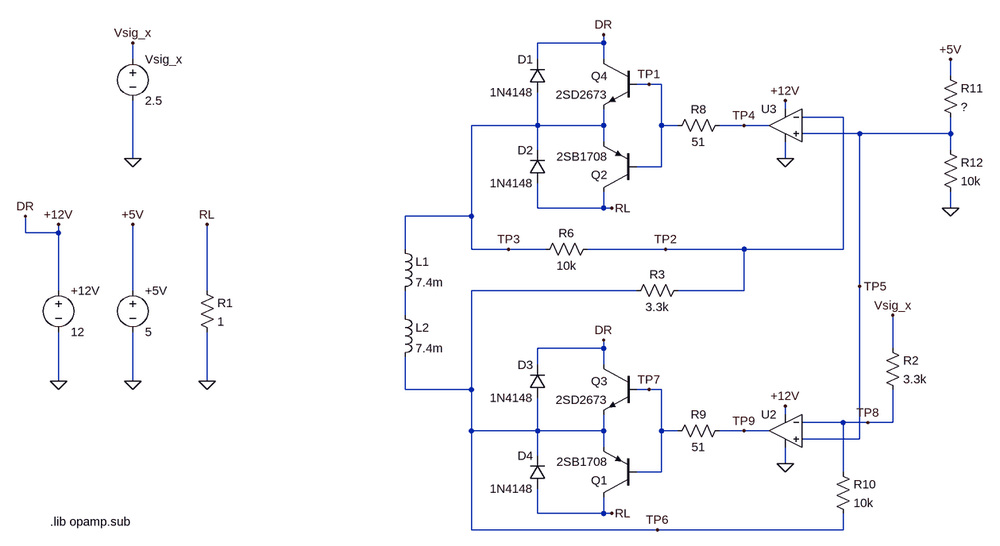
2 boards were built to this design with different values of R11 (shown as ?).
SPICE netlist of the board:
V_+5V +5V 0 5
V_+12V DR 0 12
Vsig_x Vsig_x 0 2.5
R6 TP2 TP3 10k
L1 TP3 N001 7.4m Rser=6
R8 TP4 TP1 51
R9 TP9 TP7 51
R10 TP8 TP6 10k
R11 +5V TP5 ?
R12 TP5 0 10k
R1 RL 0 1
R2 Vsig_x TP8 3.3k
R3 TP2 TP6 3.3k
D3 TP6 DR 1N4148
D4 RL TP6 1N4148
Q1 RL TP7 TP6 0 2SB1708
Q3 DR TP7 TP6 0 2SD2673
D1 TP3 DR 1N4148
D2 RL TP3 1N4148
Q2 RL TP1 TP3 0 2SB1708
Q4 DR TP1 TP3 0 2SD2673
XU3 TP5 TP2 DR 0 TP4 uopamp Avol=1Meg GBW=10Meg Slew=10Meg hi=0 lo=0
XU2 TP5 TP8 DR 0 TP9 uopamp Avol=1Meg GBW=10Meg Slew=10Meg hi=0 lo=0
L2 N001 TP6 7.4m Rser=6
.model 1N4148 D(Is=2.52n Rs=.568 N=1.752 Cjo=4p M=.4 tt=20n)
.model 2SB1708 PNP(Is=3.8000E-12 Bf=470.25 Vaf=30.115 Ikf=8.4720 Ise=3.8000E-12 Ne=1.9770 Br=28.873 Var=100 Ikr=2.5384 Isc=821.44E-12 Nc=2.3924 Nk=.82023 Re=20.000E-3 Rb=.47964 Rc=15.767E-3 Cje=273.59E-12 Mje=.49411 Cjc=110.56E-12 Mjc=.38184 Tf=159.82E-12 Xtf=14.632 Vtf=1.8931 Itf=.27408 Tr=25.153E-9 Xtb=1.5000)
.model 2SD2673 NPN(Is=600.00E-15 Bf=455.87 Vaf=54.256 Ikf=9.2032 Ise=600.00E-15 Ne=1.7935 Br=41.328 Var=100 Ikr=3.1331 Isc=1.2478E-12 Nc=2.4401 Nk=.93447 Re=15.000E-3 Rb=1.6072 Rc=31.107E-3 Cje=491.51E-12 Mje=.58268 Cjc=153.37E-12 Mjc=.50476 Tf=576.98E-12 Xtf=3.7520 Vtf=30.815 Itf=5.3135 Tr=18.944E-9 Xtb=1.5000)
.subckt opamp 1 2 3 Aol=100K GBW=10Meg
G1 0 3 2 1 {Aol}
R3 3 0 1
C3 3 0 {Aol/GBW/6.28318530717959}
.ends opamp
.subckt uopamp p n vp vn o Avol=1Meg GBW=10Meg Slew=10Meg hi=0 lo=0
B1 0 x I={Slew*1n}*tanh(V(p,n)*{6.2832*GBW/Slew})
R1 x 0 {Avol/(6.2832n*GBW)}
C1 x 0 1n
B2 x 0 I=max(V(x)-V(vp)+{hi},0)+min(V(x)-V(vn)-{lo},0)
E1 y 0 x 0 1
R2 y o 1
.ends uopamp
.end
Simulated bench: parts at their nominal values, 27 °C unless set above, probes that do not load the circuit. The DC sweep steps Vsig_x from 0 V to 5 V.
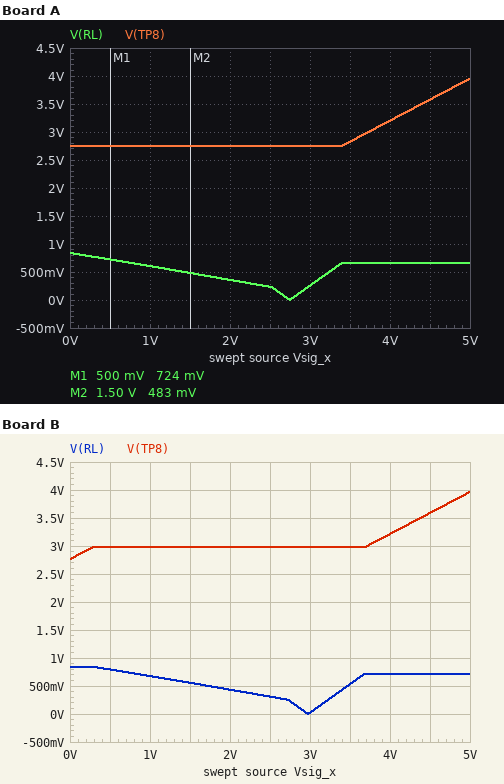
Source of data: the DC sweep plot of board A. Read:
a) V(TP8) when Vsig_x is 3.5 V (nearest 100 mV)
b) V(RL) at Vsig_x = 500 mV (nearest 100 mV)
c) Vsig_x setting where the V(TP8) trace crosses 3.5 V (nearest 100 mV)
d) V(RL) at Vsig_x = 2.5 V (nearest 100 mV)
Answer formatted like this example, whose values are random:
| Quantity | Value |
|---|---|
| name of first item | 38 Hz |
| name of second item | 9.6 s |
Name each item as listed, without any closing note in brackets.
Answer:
| Quantity | Value |
|---|---|
| V(TP8) when Vsig_x is 3.5 V | 2.8 V |
| V(RL) at Vsig_x = 500 mV | 700 mV |
| Vsig_x setting where the V(TP8) trace crosses 3.5 V | 4.4 V |
| V(RL) at Vsig_x = 2.5 V | 200 mV |
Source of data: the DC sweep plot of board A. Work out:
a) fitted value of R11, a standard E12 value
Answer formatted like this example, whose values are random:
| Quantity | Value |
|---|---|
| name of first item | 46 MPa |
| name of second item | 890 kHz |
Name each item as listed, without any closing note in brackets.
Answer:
| Quantity | Value |
|---|---|
| fitted value of R11, a standard E12 value | 8.2 kΩ |
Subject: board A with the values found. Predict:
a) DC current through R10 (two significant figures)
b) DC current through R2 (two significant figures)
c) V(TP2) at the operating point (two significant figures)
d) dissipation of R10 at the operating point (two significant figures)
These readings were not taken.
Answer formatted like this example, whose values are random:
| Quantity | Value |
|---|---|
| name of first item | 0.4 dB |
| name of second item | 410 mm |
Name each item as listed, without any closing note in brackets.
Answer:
| Quantity | Value |
|---|---|
| DC current through R10 | 75 µA |
| DC current through R2 | 75 µA |
| V(TP2) at the operating point | 2.8 V |
| dissipation of R10 at the operating point | 56 µW |
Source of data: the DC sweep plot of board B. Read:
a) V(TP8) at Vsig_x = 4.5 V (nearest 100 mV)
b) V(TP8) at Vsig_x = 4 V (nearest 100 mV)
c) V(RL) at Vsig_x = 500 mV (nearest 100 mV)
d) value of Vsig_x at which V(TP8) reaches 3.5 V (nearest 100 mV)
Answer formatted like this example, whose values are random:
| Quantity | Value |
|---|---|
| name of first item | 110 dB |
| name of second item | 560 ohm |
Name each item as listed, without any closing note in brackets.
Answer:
| Quantity | Value |
|---|---|
| V(TP8) at Vsig_x = 4.5 V | 3.6 V |
| V(TP8) at Vsig_x = 4 V | 3.2 V |
| V(RL) at Vsig_x = 500 mV | 800 mV |
| value of Vsig_x at which V(TP8) reaches 3.5 V | 4.4 V |
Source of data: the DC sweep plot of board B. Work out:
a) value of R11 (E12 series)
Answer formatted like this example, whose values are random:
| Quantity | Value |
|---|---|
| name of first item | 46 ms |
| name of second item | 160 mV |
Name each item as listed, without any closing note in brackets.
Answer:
| Quantity | Value |
|---|---|
| value of R11 | 6.8 kΩ |
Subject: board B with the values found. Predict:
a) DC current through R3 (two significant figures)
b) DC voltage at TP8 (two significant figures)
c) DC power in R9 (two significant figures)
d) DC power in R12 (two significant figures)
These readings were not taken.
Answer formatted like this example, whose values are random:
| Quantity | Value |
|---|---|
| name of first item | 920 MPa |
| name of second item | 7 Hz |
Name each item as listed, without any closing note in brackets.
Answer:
| Quantity | Value |
|---|---|
| DC current through R3 | 280 µA |
| DC voltage at TP8 | 3.0 V |
| DC power in R9 | 21 µW |
| DC power in R12 | 890 µW |
